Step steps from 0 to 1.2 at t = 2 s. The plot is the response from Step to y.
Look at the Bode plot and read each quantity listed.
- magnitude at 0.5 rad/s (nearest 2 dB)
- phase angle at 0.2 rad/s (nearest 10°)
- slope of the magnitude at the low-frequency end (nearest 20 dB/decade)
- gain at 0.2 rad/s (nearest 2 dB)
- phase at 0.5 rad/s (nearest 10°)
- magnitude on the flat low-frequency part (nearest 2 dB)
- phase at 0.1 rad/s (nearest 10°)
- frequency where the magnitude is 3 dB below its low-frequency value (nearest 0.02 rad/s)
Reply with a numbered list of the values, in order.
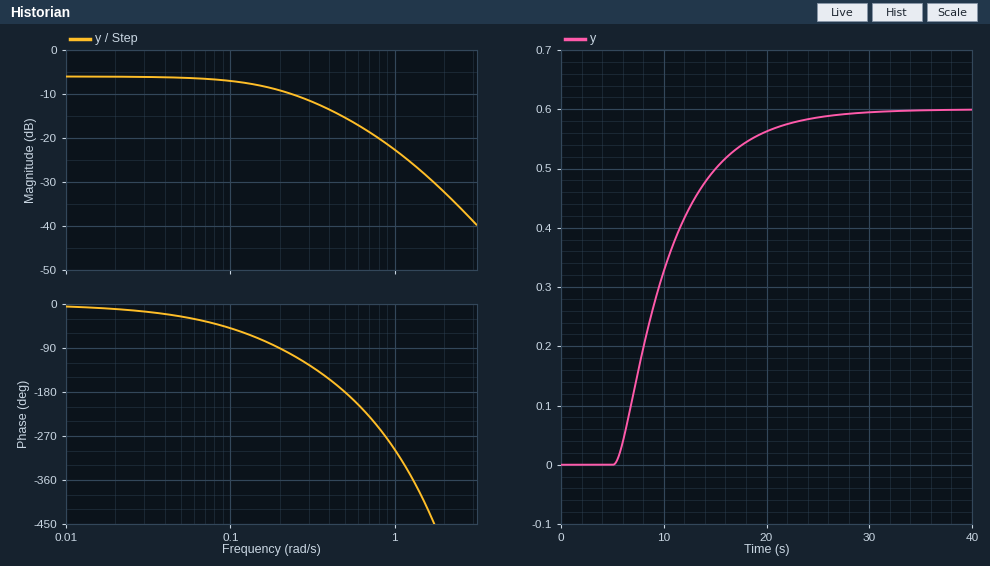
1. -16 dB
2. -90°
3. 0 dB/decade
4. -10 dB
5. -180°
6. -6 dB
7. -50°
8. 0.20 rad/s
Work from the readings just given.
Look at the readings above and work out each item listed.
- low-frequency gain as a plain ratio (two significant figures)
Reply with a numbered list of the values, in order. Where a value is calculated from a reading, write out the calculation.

1. 10^(-6 / 20) = 0.50
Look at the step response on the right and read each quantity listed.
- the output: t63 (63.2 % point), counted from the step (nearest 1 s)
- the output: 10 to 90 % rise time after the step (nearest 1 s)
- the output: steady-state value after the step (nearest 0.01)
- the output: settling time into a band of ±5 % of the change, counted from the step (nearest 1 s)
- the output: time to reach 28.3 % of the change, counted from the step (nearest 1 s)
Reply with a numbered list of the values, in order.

1. 9 s
2. 11 s
3. 0.60
4. 19 s
5. 6 s
